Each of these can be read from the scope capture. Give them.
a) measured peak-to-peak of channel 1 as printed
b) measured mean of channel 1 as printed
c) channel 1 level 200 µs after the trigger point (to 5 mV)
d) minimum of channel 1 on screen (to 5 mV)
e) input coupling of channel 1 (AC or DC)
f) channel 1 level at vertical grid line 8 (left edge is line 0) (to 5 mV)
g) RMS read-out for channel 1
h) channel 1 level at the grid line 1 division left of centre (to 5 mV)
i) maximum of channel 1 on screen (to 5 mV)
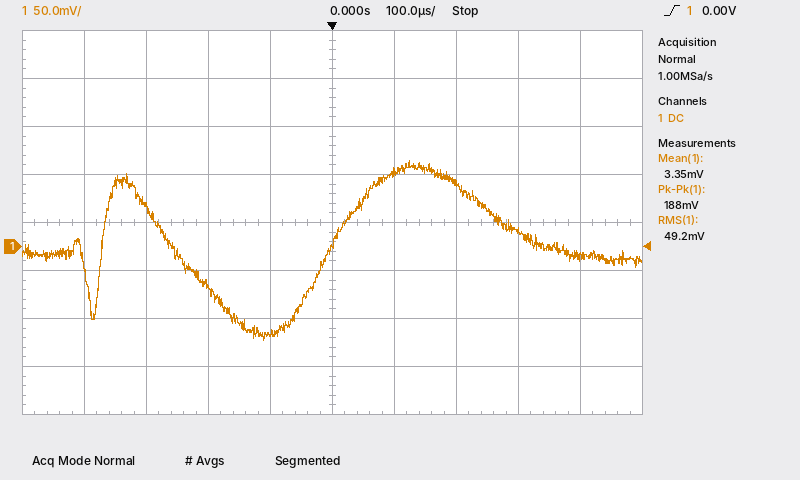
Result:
188 mV
3.35 mV
65 mV
-100 mV
DC
15 mV
49.2 mV
-90 mV
90 mV
